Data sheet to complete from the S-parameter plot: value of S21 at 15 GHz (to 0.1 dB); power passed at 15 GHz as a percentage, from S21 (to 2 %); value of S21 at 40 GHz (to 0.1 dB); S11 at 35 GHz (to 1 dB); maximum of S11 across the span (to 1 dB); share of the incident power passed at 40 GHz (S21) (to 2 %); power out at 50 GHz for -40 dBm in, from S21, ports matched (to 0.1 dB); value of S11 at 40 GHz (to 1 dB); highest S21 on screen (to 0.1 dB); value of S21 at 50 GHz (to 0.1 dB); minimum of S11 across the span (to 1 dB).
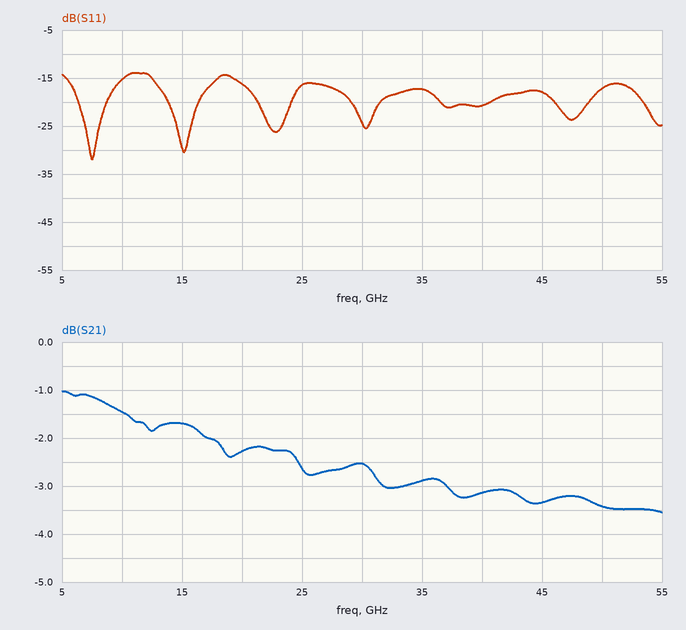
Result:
-1.7 dB
68 %
-3.1 dB
-17 dB
-14 dB
48 %
-43.4 dBm
-21 dB
-1.0 dB
-3.4 dB
-32 dB
